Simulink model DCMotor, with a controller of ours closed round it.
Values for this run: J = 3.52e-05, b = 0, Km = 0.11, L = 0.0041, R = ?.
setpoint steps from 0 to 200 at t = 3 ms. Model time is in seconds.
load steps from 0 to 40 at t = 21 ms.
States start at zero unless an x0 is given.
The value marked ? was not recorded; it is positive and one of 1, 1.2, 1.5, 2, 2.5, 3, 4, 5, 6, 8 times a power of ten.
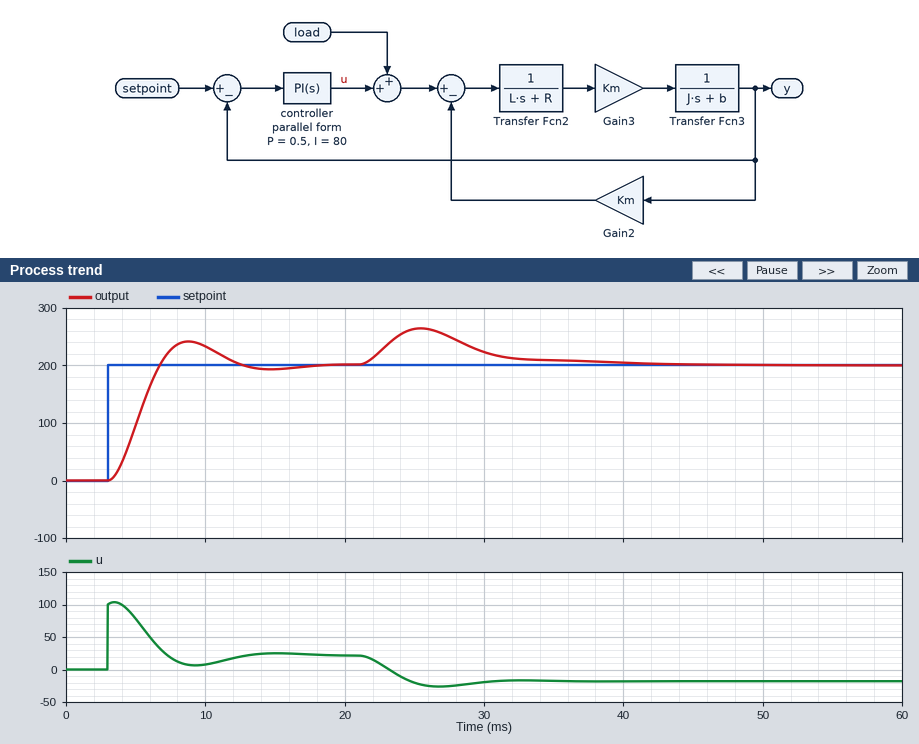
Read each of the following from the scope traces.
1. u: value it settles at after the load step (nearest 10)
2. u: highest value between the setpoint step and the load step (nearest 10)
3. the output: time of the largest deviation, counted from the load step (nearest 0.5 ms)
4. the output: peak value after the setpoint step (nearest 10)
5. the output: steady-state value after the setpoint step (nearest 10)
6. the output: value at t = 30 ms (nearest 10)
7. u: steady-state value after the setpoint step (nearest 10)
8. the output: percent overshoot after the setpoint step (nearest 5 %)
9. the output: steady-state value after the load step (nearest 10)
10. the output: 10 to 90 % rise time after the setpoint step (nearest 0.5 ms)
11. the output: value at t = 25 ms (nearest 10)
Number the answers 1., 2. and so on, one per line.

1. -20
2. 100
3. 4.5 ms
4. 240
5. 200
6. 220
7. 20
8. 20 %
9. 200
10. 2.5 ms
11. 260
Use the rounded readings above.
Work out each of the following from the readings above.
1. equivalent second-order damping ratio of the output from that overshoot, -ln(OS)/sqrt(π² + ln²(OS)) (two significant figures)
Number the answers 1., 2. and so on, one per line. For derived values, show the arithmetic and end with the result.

1. ln(0.2) = -1.609; 1.609 / sqrt(9.870 + 2.590) = 0.46
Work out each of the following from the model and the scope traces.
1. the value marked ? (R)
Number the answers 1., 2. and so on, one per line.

1. 3
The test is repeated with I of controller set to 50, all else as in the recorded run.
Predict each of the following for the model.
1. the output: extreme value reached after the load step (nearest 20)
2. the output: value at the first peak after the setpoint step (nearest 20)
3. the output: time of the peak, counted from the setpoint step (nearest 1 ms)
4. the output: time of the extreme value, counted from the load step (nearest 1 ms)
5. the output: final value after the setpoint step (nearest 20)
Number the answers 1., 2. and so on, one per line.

1. 260
2. 220
3. 6 ms
4. 5 ms
5. 200
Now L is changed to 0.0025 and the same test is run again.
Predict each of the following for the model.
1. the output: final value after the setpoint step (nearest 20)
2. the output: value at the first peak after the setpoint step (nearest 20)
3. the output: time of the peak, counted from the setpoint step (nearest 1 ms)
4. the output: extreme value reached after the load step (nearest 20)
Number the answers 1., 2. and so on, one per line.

1. 200
2. 220
3. 5 ms
4. 260
